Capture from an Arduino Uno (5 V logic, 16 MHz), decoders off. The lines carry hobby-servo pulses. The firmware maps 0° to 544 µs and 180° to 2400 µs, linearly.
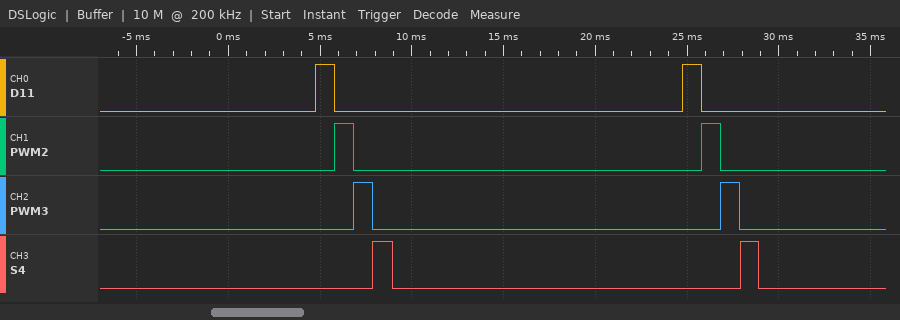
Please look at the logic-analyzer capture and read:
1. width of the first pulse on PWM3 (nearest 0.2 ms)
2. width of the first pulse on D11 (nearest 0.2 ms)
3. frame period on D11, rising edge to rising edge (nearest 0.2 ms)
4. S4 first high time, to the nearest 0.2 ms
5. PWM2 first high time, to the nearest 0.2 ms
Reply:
1.0 ms
1.0 ms
20.0 ms
1.0 ms
1.0 ms
